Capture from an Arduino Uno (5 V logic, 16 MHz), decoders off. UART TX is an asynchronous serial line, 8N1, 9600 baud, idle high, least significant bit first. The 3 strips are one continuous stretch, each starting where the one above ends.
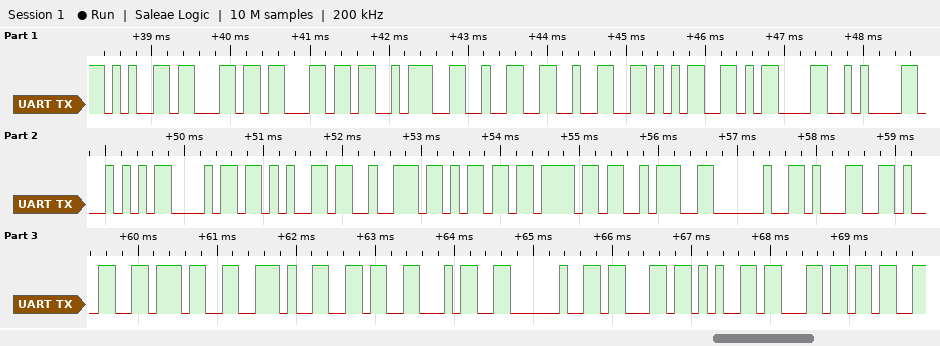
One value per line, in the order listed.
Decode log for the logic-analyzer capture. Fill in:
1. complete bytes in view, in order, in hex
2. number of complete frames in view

65 6C 6C 3A 32 32 35 0D 0A 54 68 65 72 6D 6F 3A 20 31 31 37 2E 36 34 20 63 65 6C
27
